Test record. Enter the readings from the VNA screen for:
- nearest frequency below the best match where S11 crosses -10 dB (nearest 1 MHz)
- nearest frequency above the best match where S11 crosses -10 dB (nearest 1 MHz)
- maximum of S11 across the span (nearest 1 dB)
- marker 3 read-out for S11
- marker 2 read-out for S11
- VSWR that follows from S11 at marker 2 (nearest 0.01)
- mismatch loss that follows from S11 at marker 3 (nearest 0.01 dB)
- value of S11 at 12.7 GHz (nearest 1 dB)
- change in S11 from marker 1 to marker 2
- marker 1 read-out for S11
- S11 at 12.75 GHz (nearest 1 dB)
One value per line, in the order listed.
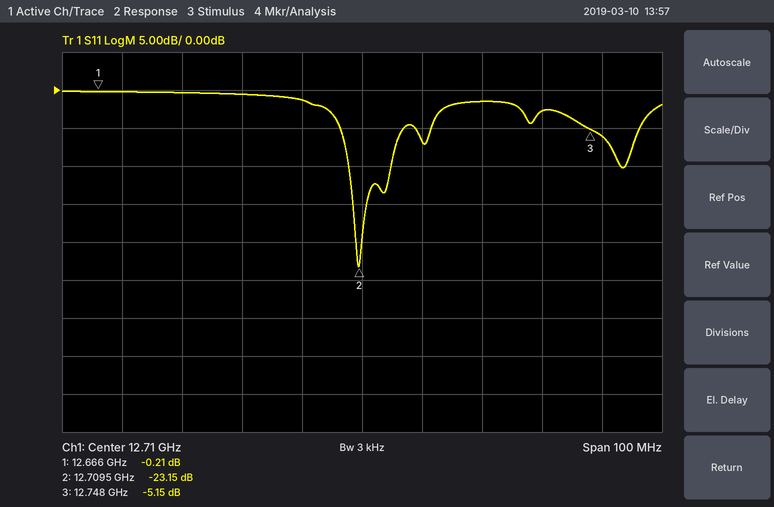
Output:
12.708 GHz
12.715 GHz
0 dB
-5.15 dB
-23.15 dB
1.15
1.58 dB
-1 dB
-22.94 dB
-0.21 dB
-6 dB
